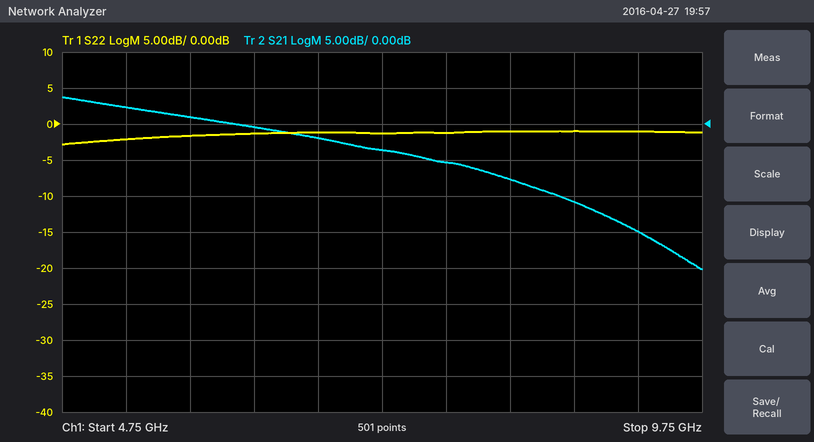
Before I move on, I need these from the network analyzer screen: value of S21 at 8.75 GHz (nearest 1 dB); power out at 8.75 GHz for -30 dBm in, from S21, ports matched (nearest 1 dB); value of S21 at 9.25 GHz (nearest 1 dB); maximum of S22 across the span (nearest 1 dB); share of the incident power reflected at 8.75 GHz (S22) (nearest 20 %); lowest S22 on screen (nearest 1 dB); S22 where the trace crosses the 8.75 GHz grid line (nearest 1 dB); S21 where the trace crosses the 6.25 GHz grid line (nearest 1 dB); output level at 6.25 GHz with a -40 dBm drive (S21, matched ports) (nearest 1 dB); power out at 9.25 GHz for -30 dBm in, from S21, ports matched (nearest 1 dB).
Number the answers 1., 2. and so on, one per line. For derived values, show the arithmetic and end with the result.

1. -11 dB
2. -30 dBm + (-11 dB) = -41 dBm
3. -15 dB
4. -1 dB
5. 10^(-1/10) ≈ 79.4 %, so 80 % to the nearest 20 %
6. -3 dB
7. -1 dB
8. 0 dB
9. -40 dBm + (0 dB) = -40 dBm
10. -30 dBm + (-15 dB) = -45 dBm
